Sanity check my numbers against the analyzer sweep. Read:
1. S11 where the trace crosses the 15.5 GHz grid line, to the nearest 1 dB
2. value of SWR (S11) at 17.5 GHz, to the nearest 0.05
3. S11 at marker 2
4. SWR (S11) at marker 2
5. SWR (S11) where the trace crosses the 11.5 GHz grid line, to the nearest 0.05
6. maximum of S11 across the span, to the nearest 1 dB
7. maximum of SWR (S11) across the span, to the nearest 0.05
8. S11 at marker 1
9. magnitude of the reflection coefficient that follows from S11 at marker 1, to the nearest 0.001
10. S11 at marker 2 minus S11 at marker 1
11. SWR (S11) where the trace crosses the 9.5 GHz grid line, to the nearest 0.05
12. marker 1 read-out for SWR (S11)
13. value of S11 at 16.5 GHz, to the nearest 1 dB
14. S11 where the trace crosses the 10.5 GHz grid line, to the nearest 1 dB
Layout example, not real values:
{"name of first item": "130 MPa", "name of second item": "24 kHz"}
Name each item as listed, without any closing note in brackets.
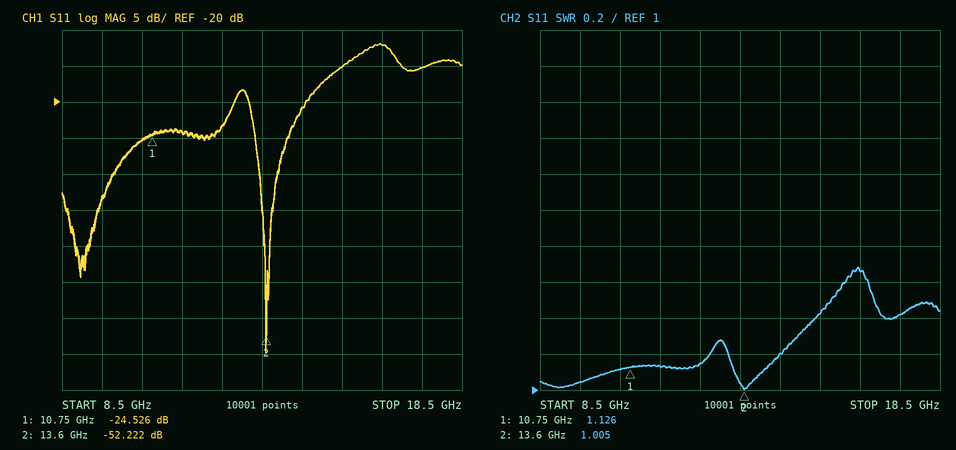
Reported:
{"S11 where the trace crosses the 15.5 GHz grid line, to the nearest 1 dB": "-15 dB", "value of SWR (S11) at 17.5 GHz, to the nearest 0.05": "1.40", "S11 at marker 2": "-52.222 dB", "SWR (S11) at marker 2": "1.005", "SWR (S11) where the trace crosses the 11.5 GHz grid line, to the nearest 0.05": "1.15", "maximum of S11 across the span, to the nearest 1 dB": "-12 dB", "maximum of SWR (S11) across the span, to the nearest 0.05": "1.70", "S11 at marker 1": "-24.526 dB", "magnitude of the reflection coefficient that follows from S11 at marker 1, to the nearest 0.001": "0.059", "S11 at marker 2 minus S11 at marker 1": "-27.696 dB", "SWR (S11) where the trace crosses the 9.5 GHz grid line, to the nearest 0.05": "1.05", "marker 1 read-out for SWR": "1.126", "value of S11 at 16.5 GHz, to the nearest 1 dB": "-12 dB", "S11 where the trace crosses the 10.5 GHz grid line, to the nearest 1 dB": "-25 dB"}
